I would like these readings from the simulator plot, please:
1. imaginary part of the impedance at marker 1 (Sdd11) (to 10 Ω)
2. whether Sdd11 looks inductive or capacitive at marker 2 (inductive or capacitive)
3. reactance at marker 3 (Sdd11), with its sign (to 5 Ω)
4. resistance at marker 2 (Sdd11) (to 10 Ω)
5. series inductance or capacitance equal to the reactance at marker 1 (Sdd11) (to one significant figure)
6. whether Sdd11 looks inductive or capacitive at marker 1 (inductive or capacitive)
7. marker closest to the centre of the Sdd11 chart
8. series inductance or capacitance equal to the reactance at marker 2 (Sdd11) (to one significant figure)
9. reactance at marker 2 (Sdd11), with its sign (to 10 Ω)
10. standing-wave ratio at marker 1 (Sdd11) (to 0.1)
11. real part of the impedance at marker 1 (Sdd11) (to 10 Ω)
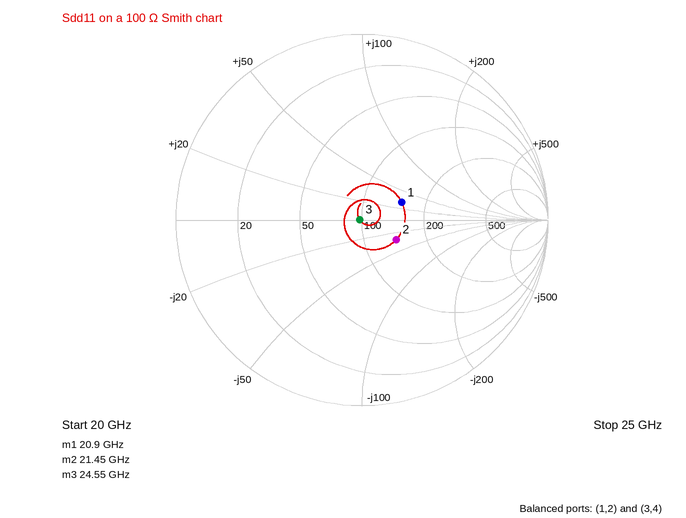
+30 Ω
capacitive
0 Ω
140 Ω
200 pH
inductive
marker 3
200 fF
-30 Ω
1.6
150 Ω
